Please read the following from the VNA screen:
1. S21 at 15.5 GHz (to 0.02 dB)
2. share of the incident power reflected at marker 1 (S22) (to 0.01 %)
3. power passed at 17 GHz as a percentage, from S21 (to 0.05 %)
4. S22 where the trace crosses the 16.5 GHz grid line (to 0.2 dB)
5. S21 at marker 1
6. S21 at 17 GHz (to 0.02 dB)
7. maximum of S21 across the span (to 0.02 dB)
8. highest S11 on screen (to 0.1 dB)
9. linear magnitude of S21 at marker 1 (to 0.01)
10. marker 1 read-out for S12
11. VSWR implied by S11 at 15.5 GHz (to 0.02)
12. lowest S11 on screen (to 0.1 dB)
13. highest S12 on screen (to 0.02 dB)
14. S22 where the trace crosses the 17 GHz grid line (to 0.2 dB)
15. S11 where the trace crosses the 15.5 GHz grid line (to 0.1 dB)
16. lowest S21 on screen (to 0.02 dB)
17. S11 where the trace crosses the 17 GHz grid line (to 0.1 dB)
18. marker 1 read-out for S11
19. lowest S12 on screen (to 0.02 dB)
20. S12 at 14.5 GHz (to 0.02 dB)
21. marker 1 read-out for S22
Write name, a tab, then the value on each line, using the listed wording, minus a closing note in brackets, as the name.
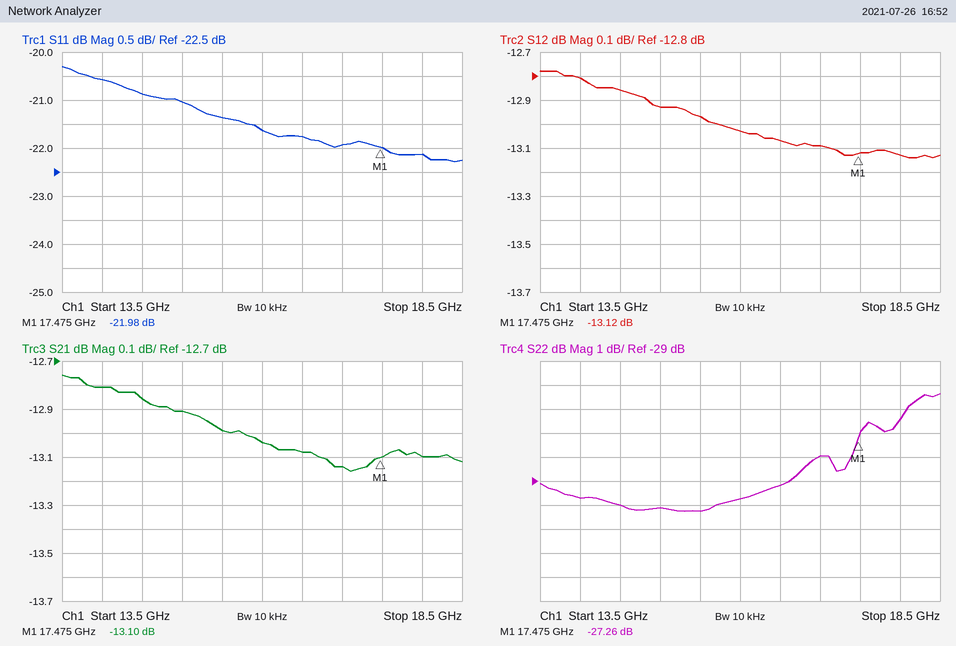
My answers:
S21 at 15.5 GHz	-12.98 dB
share of the incident power reflected at marker 1 (S22)	0.19 %
power passed at 17 GHz as a percentage, from S21	4.85 %
S22 where the trace crosses the 16.5 GHz grid line	-29.2 dB
S21 at marker 1	-13.10 dB
S21 at 17 GHz	-13.14 dB
maximum of S21 across the span	-12.76 dB
highest S11 on screen	-20.3 dB
linear magnitude of S21 at marker 1	0.22
marker 1 read-out for S12	-13.12 dB
VSWR implied by S11 at 15.5 GHz	1.18
lowest S11 on screen	-22.3 dB
highest S12 on screen	-12.78 dB
S22 where the trace crosses the 17 GHz grid line	-28.0 dB
S11 where the trace crosses the 15.5 GHz grid line	-21.4 dB
lowest S21 on screen	-13.16 dB
S11 where the trace crosses the 17 GHz grid line	-21.9 dB
marker 1 read-out for S11	-21.98 dB
lowest S12 on screen	-13.14 dB
S12 at 14.5 GHz	-12.86 dB
marker 1 read-out for S22	-27.26 dB
